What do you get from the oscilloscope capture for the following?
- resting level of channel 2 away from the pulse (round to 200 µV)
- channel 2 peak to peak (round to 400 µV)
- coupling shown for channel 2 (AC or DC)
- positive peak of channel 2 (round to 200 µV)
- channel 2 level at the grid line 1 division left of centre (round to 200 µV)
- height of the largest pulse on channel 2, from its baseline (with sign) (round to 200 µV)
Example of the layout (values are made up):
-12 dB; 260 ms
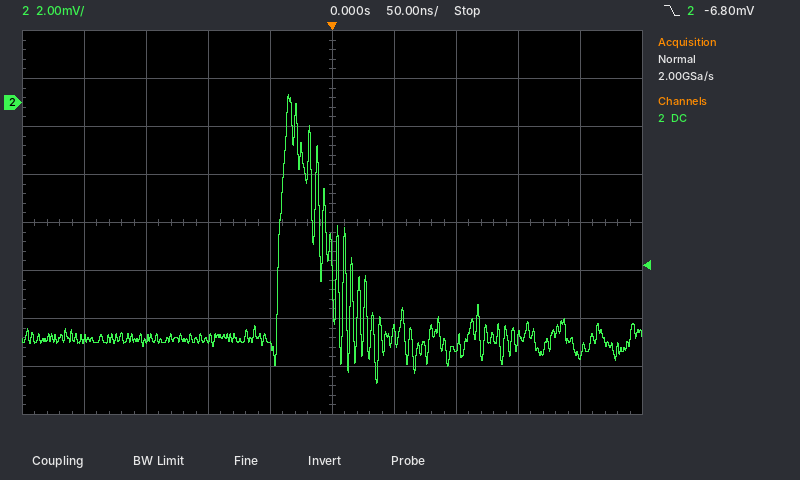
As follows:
-9.8 mV; 12.0 mV; DC; 400 µV; -10.2 mV; +10.2 mV
